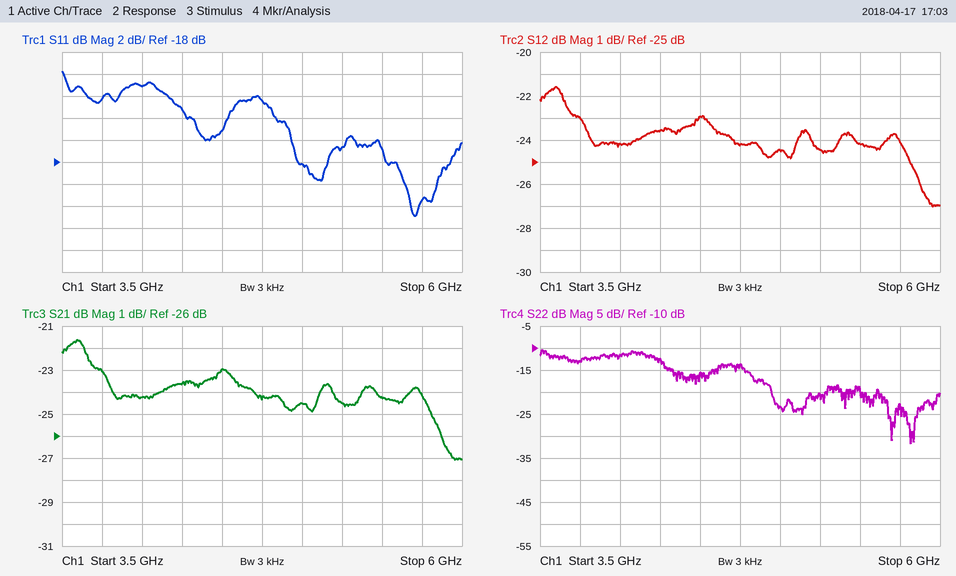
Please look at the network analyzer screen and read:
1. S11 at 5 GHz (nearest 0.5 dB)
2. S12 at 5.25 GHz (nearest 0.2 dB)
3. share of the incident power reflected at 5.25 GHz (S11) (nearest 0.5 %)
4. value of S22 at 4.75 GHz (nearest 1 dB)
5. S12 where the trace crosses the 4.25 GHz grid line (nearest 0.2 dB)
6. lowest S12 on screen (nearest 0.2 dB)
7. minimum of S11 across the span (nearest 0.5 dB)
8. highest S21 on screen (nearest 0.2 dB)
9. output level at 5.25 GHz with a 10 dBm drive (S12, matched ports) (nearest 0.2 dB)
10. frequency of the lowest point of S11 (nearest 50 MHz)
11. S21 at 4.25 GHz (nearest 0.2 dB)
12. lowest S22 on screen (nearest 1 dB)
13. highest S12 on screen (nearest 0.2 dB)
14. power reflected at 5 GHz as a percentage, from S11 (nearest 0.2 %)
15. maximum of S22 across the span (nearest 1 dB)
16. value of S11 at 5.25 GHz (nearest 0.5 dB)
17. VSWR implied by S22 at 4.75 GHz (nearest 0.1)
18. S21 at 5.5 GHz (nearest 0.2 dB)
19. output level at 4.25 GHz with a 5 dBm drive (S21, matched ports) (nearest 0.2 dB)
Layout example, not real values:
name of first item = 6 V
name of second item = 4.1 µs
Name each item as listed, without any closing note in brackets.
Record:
S11 at 5 GHz = -18.0 dB
S12 at 5.25 GHz = -24.4 dB
share of the incident power reflected at 5.25 GHz (S11) = 2.0 %
value of S22 at 4.75 GHz = -14 dB
S12 where the trace crosses the 4.25 GHz grid line = -23.6 dB
lowest S12 on screen = -27.0 dB
minimum of S11 across the span = -23.0 dB
highest S21 on screen = -21.6 dB
output level at 5.25 GHz with a 10 dBm drive (S12, matched ports) = -14.4 dBm
frequency of the lowest point of S11 = 5.70 GHz
S21 at 4.25 GHz = -23.6 dB
lowest S22 on screen = -32 dB
highest S12 on screen = -21.6 dB
power reflected at 5 GHz as a percentage, from S11 = 1.6 %
maximum of S22 across the span = -10 dB
value of S11 at 5.25 GHz = -16.5 dB
VSWR implied by S22 at 4.75 GHz = 1.5
S21 at 5.5 GHz = -24.2 dB
output level at 4.25 GHz with a 5 dBm drive (S21, matched ports) = -18.6 dBm
